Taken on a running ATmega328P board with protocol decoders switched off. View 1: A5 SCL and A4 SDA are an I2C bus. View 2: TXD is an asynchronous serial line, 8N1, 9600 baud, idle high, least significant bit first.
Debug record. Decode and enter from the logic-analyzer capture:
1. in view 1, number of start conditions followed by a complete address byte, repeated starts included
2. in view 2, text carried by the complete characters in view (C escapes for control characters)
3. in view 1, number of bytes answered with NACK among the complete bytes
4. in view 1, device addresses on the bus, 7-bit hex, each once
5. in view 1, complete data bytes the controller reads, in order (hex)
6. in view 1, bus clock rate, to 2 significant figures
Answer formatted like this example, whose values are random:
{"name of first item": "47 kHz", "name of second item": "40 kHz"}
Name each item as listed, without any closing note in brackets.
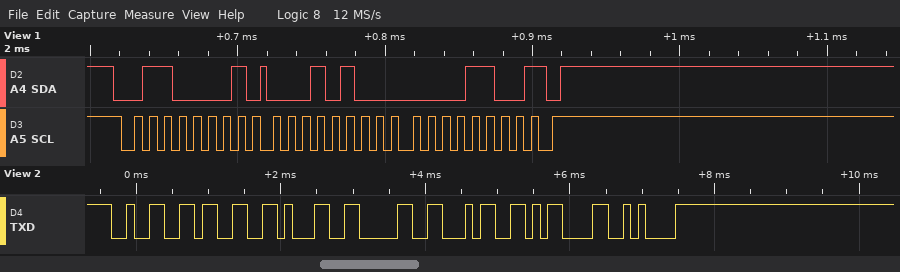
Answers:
{"in view 1, number of start conditions followed by a complete address byte, repeated starts included": "1", "in view 2, text carried by the complete characters in view": "\"23104\\r\\n\"", "in view 1, number of bytes answered with NACK among the complete bytes": "1", "in view 1, device addresses on the bus, 7-bit hex, each once": "0x30", "in view 1, complete data bytes the controller reads, in order": "14 0C", "in view 1, bus clock rate, to 2 significant figures": "100 kHz"}
